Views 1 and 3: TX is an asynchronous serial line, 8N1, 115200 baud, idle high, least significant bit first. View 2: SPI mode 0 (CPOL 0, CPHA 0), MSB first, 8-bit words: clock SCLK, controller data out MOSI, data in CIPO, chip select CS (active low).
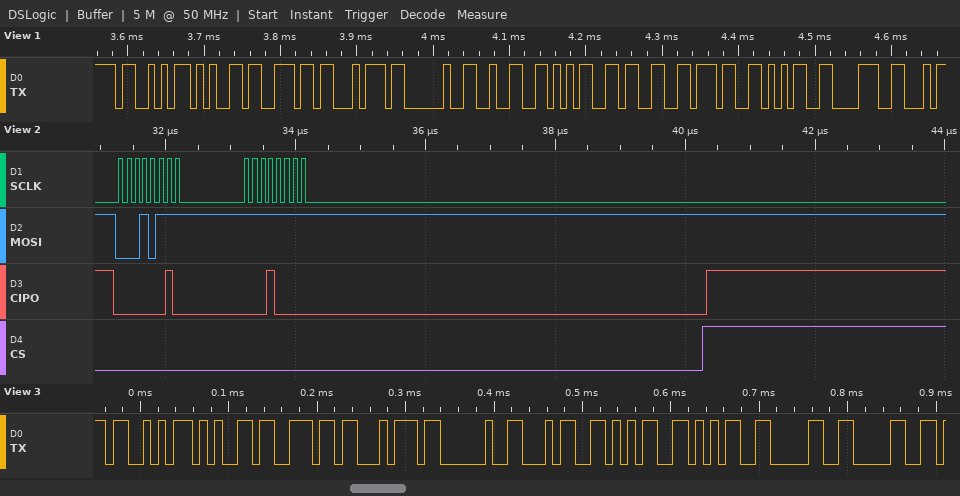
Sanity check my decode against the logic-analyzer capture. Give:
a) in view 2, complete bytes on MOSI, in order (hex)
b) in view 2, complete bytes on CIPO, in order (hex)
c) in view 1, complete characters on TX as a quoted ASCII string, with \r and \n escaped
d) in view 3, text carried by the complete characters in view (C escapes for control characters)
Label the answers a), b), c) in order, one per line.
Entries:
a) 17 FF
b) 02 10
c) "Sent 253758"
d) "Sent 45500"
